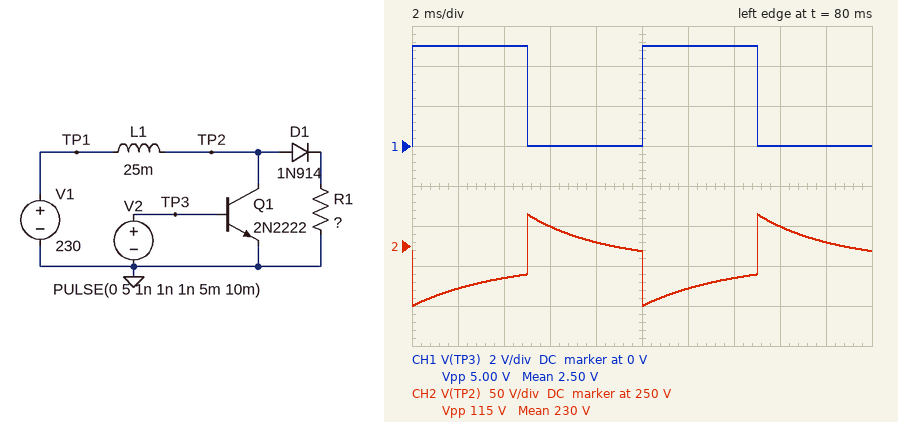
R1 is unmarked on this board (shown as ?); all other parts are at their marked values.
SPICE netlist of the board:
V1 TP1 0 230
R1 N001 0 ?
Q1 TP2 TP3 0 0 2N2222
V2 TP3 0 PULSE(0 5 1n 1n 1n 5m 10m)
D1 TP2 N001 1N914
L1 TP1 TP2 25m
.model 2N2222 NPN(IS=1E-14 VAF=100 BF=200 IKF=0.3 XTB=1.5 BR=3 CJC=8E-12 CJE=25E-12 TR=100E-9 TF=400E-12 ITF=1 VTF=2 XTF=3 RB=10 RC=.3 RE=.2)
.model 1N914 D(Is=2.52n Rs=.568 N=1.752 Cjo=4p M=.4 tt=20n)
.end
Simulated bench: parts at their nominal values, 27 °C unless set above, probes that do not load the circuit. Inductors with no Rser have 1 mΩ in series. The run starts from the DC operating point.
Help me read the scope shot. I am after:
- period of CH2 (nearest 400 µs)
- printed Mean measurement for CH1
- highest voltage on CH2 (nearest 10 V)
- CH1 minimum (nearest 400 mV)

10.0 ms
2.50 V
290 V
0 V
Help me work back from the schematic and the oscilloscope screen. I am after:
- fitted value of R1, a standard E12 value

6.8 Ω
